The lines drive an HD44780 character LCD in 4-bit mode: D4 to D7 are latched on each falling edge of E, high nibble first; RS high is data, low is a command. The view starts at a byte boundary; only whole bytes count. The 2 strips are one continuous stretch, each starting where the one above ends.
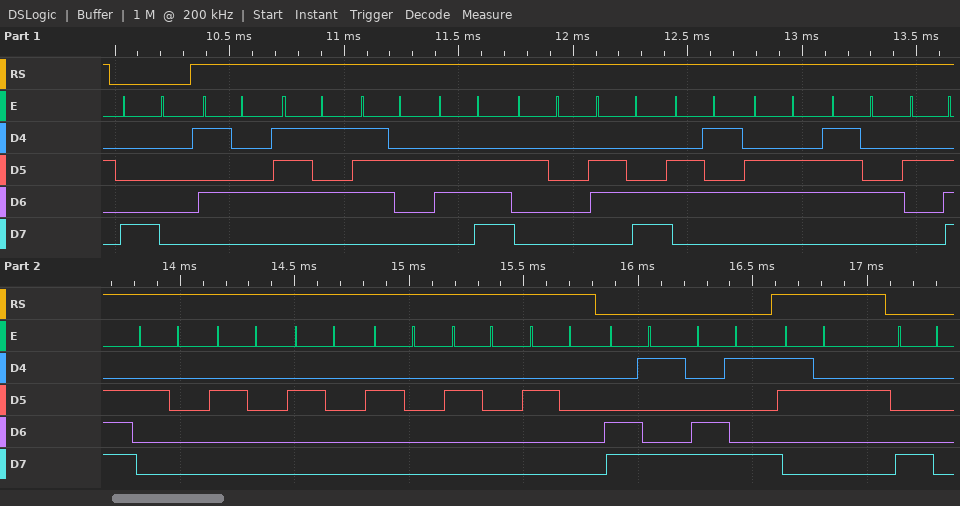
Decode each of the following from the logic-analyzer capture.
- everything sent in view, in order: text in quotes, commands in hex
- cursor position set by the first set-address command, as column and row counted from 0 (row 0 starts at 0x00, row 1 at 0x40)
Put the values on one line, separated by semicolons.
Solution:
0x80 "Turn left.      " 0xC9 0xC9 "2" 0x80; column 0, row 0
